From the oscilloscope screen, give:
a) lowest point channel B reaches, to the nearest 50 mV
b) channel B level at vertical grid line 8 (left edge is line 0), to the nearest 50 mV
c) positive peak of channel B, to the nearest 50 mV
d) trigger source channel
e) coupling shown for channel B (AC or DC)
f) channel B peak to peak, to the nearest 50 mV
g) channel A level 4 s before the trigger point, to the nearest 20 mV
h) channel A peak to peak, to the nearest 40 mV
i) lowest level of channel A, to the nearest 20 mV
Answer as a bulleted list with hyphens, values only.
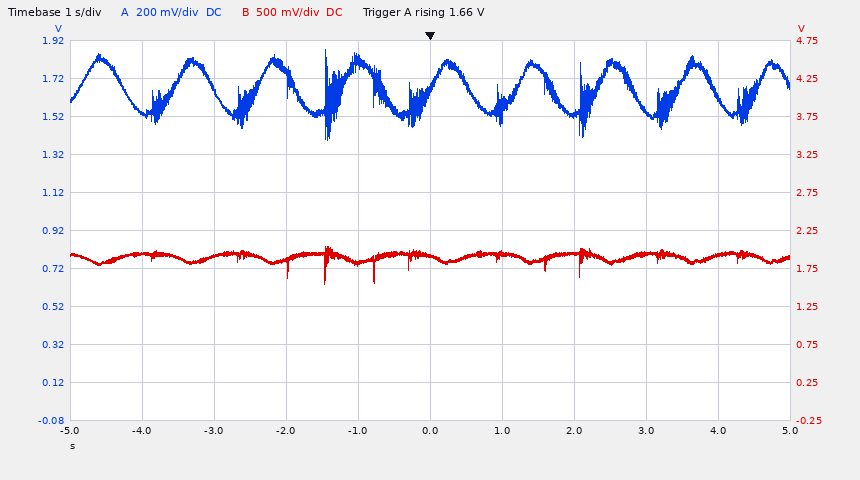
- 1.55 V
- 1.95 V
- 2.05 V
- channel A
- DC
- 500 mV
- 1.54 V
- 480 mV
- 1.40 V
